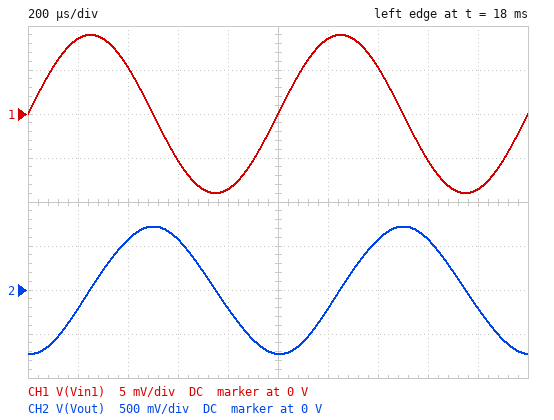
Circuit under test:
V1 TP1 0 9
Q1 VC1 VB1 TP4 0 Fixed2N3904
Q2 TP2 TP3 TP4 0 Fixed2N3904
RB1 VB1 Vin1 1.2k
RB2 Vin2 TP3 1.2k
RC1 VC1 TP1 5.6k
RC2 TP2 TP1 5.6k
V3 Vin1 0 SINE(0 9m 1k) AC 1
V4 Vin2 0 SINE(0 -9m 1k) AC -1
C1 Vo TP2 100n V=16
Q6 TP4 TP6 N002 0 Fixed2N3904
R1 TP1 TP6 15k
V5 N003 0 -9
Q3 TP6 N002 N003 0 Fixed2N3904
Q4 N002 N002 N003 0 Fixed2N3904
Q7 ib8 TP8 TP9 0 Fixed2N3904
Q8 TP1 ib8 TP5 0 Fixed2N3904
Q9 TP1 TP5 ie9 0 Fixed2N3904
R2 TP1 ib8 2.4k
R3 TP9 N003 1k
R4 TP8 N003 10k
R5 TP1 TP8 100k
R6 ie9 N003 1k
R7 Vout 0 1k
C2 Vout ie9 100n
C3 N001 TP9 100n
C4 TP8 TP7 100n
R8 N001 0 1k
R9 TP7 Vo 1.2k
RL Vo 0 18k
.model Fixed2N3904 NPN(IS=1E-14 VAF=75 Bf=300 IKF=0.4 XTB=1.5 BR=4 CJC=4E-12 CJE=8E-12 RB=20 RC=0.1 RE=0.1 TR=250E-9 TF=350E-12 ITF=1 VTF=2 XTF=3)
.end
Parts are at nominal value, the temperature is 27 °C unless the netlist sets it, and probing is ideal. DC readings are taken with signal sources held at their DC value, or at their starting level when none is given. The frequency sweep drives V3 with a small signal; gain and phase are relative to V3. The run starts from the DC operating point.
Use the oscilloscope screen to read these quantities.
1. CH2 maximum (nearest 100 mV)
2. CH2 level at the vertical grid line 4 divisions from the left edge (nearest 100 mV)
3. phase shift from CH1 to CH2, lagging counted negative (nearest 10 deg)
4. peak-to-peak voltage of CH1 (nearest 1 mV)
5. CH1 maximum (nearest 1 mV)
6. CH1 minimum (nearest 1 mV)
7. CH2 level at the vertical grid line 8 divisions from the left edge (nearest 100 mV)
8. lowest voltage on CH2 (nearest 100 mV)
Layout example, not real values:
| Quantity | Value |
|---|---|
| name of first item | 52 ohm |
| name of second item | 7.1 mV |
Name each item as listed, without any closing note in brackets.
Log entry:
| Quantity | Value |
|---|---|
| CH2 maximum | 700 mV |
| CH2 level at the vertical grid line 4 divisions from the left edge | -200 mV |
| phase shift from CH1 to CH2, lagging counted negative | -90 deg |
| peak-to-peak voltage of CH1 | 18 mV |
| CH1 maximum | 9 mV |
| CH1 minimum | -9 mV |
| CH2 level at the vertical grid line 8 divisions from the left edge | 600 mV |
| lowest voltage on CH2 | -700 mV |
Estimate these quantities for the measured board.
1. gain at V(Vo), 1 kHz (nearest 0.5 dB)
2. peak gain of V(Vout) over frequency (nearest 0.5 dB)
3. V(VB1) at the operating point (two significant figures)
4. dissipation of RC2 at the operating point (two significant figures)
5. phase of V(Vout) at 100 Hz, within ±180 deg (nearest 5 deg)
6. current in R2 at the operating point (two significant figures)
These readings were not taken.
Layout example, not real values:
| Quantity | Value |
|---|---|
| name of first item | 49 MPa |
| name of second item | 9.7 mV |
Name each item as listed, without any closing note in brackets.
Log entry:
| Quantity | Value |
|---|---|
| gain at V(Vo), 1 kHz | 35.0 dB |
| peak gain of V(Vout) over frequency | 47.0 dB |
| V(VB1) at the operating point | -2.0 mV |
| dissipation of RC2 at the operating point | 1.7 mW |
| phase of V(Vout) at 100 Hz, within ±180 deg | -5 deg |
| current in R2 at the operating point | 960 µA |
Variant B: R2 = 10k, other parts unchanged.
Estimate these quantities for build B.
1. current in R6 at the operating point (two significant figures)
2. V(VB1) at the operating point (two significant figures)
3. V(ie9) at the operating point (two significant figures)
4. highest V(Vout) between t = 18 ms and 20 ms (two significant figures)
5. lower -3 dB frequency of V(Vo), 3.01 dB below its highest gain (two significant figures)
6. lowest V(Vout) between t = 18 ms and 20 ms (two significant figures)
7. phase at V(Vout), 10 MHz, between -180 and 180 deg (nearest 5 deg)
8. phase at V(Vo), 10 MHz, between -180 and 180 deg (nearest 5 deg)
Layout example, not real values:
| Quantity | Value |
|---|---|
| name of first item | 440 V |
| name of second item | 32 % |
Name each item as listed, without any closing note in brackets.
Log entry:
| Quantity | Value |
|---|---|
| current in R6 at the operating point | 7.2 mA |
| V(VB1) at the operating point | -2.0 mV |
| V(ie9) at the operating point | -1.8 V |
| highest V(Vout) between t = 18 ms and 20 ms | 3.0 V |
| lower -3 dB frequency of V(Vo), 3.01 dB below its highest gain | 71 Hz |
| lowest V(Vout) between t = 18 ms and 20 ms | -3.0 V |
| phase at V(Vout), 10 MHz, between -180 and 180 deg | 5 deg |
| phase at V(Vo), 10 MHz, between -180 and 180 deg | -75 deg |
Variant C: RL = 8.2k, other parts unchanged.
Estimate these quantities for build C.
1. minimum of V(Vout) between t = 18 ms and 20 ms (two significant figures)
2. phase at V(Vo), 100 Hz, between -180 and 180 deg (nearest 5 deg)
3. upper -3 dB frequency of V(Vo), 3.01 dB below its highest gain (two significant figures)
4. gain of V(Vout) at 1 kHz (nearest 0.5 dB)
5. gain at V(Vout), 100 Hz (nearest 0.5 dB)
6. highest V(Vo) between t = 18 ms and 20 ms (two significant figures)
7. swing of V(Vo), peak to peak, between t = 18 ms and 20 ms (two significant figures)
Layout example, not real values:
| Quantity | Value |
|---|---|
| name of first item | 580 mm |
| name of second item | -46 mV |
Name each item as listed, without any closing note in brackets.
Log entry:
| Quantity | Value |
|---|---|
| minimum of V(Vout) between t = 18 ms and 20 ms | -610 mV |
| phase at V(Vo), 100 Hz, between -180 and 180 deg | 40 deg |
| upper -3 dB frequency of V(Vo), 3.01 dB below its highest gain | 710 kHz |
| gain of V(Vout) at 1 kHz | 36.5 dB |
| gain at V(Vout), 100 Hz | 7.0 dB |
| highest V(Vo) between t = 18 ms and 20 ms | 410 mV |
| swing of V(Vo), peak to peak, between t = 18 ms and 20 ms | 820 mV |
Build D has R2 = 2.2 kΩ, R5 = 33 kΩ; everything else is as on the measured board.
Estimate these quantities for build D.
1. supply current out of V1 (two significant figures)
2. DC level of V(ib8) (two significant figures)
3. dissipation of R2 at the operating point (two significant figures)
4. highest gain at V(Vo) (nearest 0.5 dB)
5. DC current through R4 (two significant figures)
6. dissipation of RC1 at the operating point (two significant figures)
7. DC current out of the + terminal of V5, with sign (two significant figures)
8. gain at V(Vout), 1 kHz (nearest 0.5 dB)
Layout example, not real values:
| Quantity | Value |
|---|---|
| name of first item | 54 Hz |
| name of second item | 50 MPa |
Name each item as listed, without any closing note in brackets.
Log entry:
| Quantity | Value |
|---|---|
| supply current out of V1 | 15 mA |
| DC level of V(ib8) | 1.5 V |
| dissipation of R2 at the operating point | 26 mW |
| highest gain at V(Vo) | 34.5 dB |
| DC current through R4 | 410 µA |
| dissipation of RC1 at the operating point | 1.7 mW |
| DC current out of the + terminal of V5, with sign | -15 mA |
| gain at V(Vout), 1 kHz | 37.0 dB |
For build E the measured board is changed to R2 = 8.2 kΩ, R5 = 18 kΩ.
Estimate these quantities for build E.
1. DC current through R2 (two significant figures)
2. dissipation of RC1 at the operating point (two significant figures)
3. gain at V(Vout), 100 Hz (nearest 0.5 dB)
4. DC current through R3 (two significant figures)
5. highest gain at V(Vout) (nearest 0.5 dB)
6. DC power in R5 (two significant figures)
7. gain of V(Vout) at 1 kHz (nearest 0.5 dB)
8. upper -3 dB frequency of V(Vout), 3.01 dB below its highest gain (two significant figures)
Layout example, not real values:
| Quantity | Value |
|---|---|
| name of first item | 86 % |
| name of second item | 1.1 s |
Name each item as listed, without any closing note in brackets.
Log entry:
| Quantity | Value |
|---|---|
| DC current through R2 | 1.9 mA |
| dissipation of RC1 at the operating point | 1.7 mW |
| gain at V(Vout), 100 Hz | -18.0 dB |
| DC current through R3 | 2.4 mA |
| highest gain at V(Vout) | 14.5 dB |
| DC power in R5 | 12 mW |
| gain of V(Vout) at 1 kHz | 11.0 dB |
| upper -3 dB frequency of V(Vout), 3.01 dB below its highest gain | 880 kHz |
